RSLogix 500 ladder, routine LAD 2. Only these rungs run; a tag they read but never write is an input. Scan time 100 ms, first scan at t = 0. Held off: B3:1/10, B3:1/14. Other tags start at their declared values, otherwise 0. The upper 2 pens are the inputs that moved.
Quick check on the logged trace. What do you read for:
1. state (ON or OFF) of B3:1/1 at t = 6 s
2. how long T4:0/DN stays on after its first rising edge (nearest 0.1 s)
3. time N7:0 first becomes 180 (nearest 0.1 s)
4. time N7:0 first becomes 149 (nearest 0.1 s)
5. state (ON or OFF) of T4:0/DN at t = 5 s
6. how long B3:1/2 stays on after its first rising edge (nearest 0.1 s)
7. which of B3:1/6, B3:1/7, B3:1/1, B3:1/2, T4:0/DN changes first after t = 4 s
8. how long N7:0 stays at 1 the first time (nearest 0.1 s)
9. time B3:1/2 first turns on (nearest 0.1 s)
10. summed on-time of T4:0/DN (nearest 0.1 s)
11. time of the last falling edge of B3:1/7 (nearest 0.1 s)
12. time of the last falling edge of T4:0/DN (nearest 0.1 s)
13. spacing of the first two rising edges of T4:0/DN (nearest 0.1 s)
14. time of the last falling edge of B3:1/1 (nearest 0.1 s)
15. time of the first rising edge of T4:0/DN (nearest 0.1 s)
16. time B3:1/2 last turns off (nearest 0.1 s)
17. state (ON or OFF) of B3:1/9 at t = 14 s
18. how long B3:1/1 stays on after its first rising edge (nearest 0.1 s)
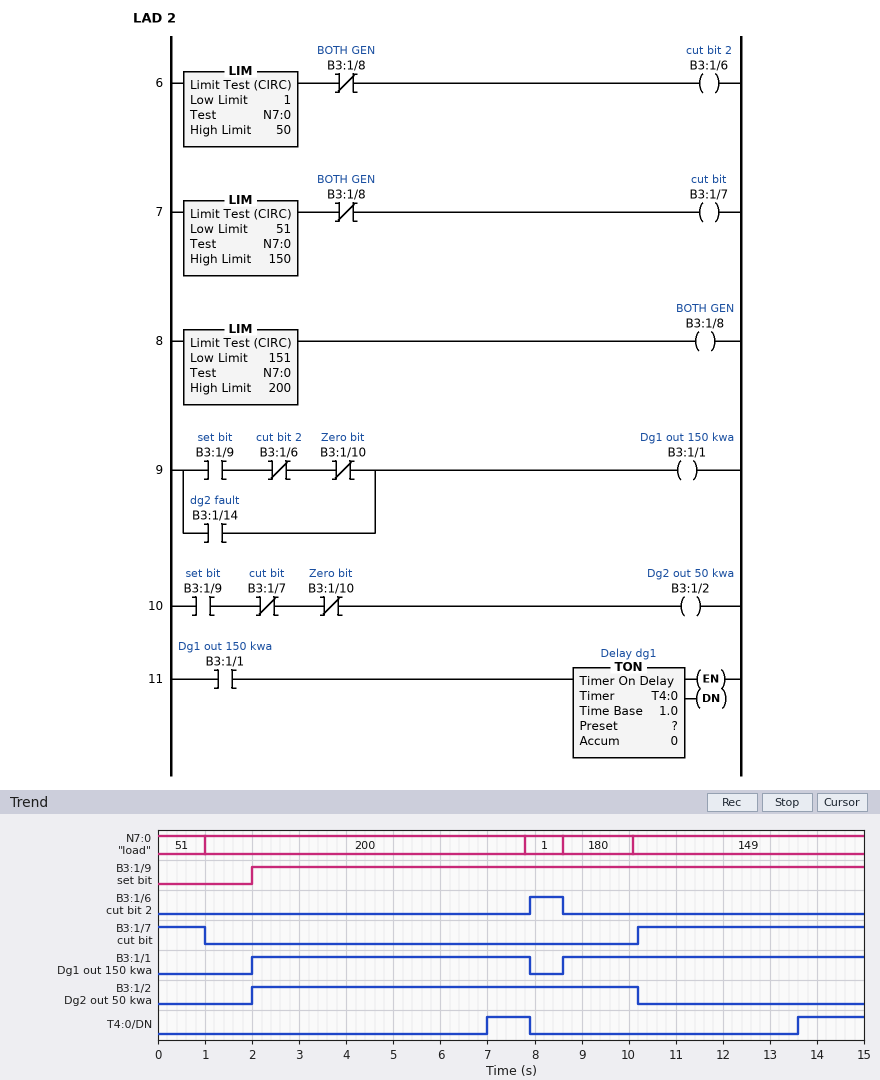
ON
0.9 s
8.6 s
10.1 s
OFF
8.2 s
T4:0/DN
0.8 s
2.0 s
2.3 s
1.0 s
7.9 s
6.6 s
7.9 s
7.0 s
10.2 s
ON
5.9 s
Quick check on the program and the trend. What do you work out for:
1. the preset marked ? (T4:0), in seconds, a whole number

5 s
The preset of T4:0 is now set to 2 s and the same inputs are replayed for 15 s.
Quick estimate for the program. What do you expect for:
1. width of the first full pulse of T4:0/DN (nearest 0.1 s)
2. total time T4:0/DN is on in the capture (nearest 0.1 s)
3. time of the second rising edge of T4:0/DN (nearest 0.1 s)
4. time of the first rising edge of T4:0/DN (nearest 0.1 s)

3.9 s
8.3 s
10.6 s
4.0 s
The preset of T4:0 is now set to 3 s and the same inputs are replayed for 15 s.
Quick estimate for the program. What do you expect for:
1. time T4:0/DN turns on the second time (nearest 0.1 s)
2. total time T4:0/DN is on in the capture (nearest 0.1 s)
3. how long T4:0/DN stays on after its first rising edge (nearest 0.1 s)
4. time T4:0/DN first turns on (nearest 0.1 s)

11.6 s
6.3 s
2.9 s
5.0 s
